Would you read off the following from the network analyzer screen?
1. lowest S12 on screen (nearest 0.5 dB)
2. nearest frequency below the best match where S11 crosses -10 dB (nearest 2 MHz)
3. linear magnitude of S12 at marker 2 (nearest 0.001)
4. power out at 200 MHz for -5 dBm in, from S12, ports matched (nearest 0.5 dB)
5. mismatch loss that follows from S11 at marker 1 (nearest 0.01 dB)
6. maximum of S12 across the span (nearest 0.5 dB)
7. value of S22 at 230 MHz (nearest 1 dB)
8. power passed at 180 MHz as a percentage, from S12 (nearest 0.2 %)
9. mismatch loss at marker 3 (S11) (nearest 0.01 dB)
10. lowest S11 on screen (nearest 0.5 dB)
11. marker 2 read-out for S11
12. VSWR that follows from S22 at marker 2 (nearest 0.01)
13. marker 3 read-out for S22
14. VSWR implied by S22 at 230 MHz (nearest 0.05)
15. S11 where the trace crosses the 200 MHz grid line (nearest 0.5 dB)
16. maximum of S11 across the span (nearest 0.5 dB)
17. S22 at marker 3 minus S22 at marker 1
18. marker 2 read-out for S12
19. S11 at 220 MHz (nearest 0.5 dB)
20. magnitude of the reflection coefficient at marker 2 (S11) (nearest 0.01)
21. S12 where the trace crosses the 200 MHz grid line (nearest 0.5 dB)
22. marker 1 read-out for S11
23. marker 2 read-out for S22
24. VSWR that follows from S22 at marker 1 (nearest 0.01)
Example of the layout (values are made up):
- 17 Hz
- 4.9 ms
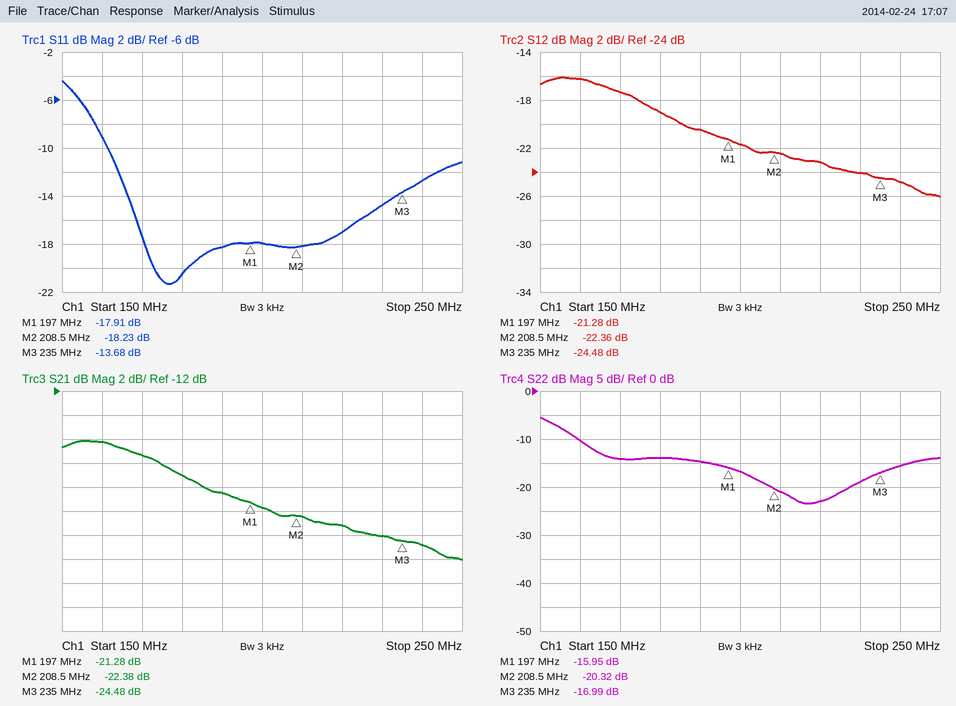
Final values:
- -26.0 dB
- 162 MHz
- 0.076
- -26.5 dBm
- 0.07 dB
- -16.0 dB
- -19 dB
- 1.2 %
- 0.19 dB
- -21.5 dB
- -18.23 dB
- 1.21
- -16.99 dB
- 1.25
- -18.0 dB
- -4.5 dB
- -1.04 dB
- -22.36 dB
- -17.0 dB
- 0.12
- -21.5 dB
- -17.91 dB
- -20.32 dB
- 1.38
